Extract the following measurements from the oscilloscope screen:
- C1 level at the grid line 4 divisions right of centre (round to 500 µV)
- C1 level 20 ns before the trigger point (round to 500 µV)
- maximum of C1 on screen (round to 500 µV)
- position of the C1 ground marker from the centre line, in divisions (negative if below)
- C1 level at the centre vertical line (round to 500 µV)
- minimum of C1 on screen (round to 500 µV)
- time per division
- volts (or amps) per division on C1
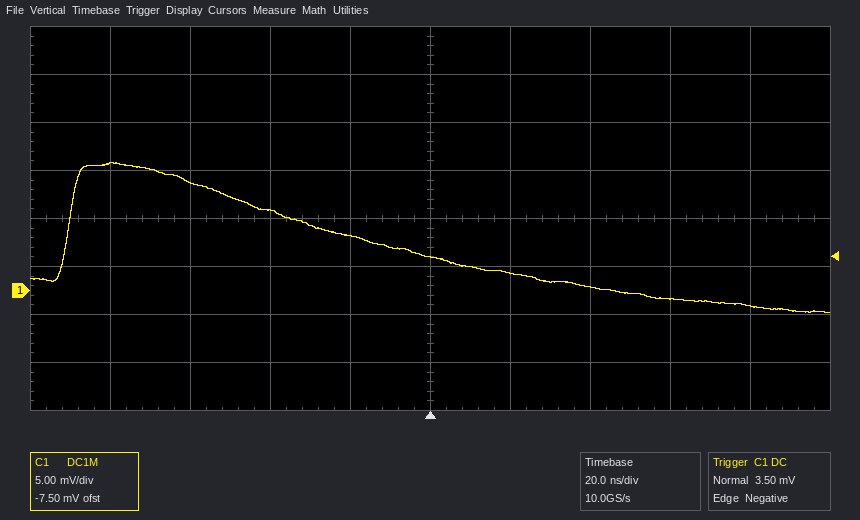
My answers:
-1.5 mV
5.5 mV
13.5 mV
-1.5 div
3.5 mV
-2.5 mV
20 ns
5 mV
